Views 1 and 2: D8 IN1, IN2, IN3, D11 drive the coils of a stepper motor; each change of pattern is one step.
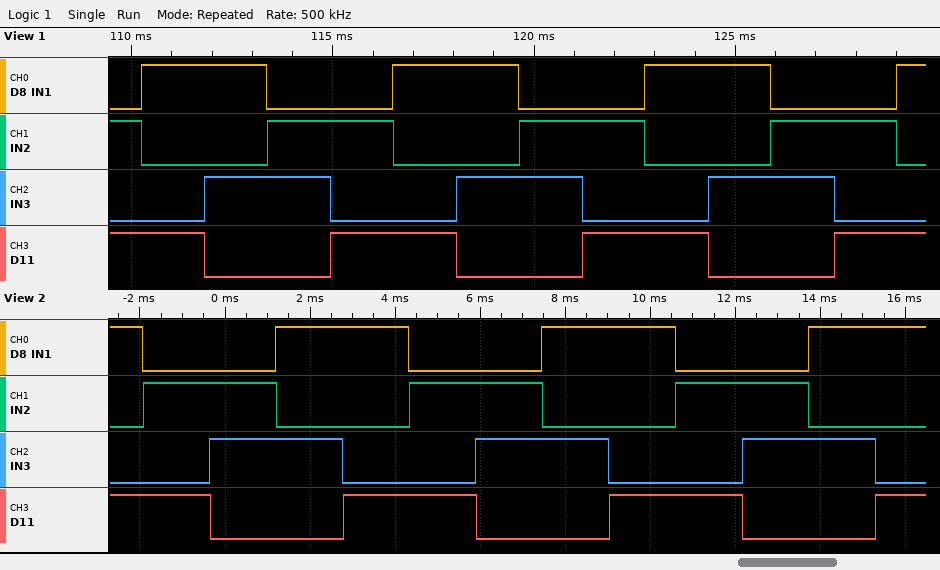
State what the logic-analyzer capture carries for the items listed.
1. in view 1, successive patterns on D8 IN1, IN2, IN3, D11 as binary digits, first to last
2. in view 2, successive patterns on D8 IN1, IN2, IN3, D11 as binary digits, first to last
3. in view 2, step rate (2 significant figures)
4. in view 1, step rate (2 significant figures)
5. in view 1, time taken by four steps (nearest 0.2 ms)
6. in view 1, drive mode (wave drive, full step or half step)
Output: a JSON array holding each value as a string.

["0101 1001 1010 0110 0101 1001 1010 0110 0101 1001 1010 0110 0101 1001", "1001 0101 0110 1010 1001 0101 0110 1010 1001 0101 0110 1010 1001", "640 steps/s", "640 steps/s", "6.2 ms", "full step"]
